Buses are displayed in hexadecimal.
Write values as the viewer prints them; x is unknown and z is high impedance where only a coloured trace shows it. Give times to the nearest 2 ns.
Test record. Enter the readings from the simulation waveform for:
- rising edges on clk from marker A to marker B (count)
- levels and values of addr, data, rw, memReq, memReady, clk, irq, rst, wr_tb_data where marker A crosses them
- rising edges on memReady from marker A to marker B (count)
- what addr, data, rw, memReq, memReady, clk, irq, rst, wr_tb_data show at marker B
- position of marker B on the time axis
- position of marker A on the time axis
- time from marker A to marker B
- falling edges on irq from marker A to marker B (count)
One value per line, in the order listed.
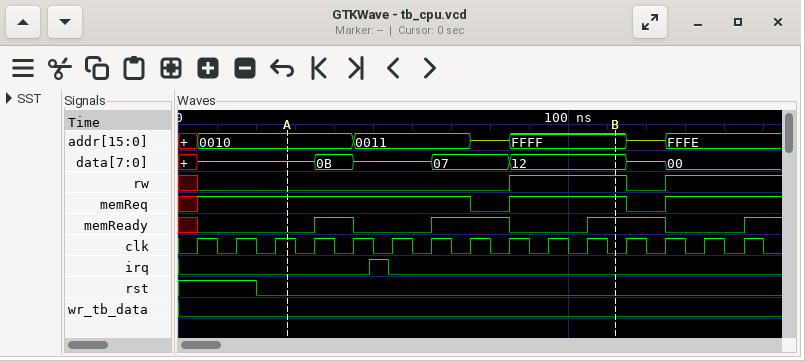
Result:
8
addr=0010, data=z, rw=0, memReq=1, memReady=0, clk=1, irq=0, rst=0, wr_tb_data=0
3
addr=FFFF, data=12, rw=1, memReq=1, memReady=1, clk=0, irq=0, rst=0, wr_tb_data=0
112 ns
28 ns
84 ns
1
